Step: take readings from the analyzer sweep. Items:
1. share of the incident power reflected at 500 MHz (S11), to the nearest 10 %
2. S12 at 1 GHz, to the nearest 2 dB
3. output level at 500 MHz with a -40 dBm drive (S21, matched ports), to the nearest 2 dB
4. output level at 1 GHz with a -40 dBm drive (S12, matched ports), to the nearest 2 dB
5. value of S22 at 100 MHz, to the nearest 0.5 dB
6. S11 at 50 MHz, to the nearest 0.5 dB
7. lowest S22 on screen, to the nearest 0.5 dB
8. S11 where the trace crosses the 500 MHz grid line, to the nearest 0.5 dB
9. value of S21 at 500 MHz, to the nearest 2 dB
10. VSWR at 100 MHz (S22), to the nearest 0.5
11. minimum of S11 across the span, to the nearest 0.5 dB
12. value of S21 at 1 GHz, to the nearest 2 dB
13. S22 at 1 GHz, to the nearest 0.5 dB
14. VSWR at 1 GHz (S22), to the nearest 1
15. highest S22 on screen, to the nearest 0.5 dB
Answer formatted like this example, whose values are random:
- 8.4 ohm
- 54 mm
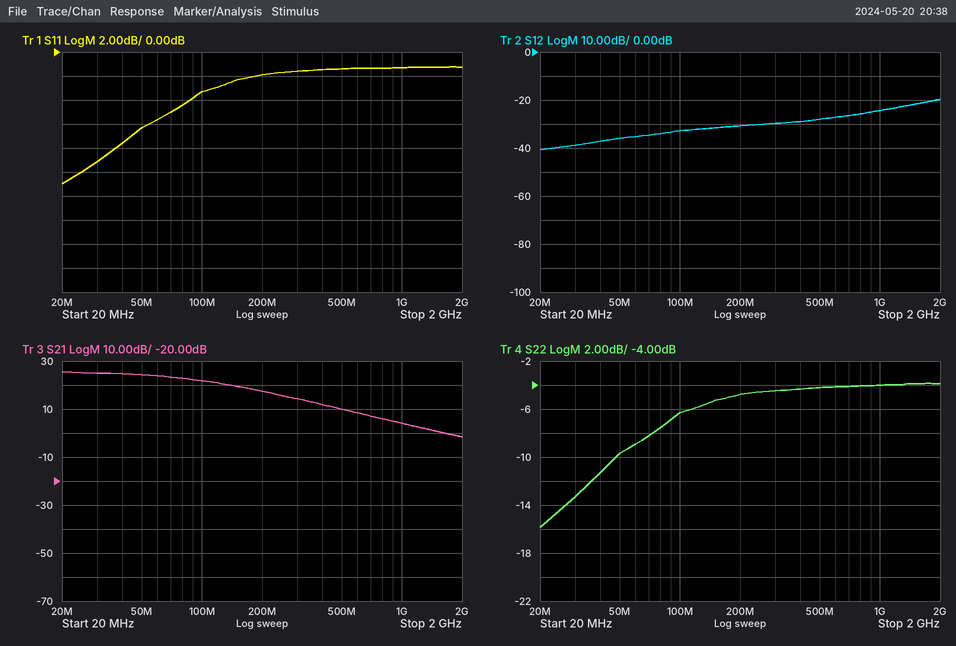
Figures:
- 70 %
- -24 dB
- -30 dBm
- -64 dBm
- -6.5 dB
- -6.5 dB
- -16.0 dB
- -1.5 dB
- 10 dB
- 3.0
- -11.0 dB
- 4 dB
- -4.0 dB
- 4
- -4.0 dB
